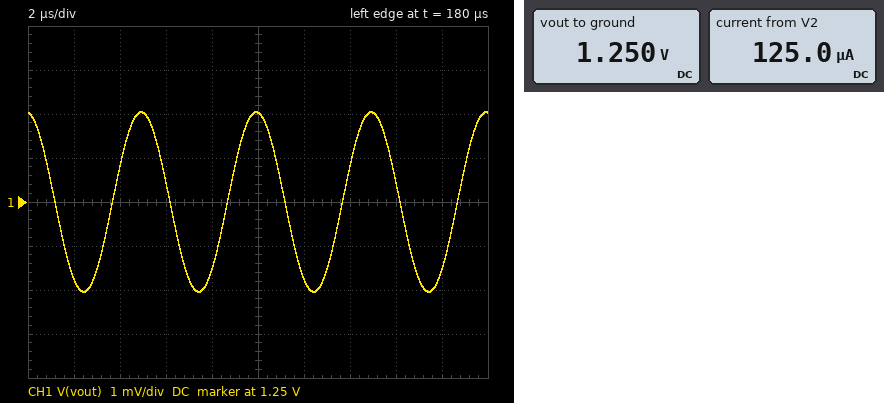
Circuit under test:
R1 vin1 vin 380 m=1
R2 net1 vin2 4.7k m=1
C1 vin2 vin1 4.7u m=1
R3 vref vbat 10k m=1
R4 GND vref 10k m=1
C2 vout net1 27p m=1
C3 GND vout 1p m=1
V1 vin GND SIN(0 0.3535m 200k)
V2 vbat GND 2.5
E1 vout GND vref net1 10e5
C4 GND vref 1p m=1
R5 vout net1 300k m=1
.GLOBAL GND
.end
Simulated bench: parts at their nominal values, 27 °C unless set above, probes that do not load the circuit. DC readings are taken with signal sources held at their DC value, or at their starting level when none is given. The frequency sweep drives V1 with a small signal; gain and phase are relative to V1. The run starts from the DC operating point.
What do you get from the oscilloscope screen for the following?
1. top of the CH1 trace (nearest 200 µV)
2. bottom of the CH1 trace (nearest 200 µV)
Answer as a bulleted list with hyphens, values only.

- 1.2520 V
- 1.2480 V
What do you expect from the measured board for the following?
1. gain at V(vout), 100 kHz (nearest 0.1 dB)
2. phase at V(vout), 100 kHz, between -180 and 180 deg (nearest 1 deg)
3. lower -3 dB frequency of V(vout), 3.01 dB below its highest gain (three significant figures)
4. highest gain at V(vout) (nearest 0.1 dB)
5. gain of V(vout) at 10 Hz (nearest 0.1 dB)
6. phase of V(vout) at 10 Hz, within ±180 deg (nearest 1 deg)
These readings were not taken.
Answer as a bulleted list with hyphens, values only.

- 21.1 dB
- 101 deg
- 6.66 Hz
- 35.4 dB
- 33.8 dB
- -146 deg
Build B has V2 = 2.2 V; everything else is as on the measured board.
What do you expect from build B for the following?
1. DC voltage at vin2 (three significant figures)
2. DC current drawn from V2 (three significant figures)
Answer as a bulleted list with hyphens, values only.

- 1.10 V
- 110 µA
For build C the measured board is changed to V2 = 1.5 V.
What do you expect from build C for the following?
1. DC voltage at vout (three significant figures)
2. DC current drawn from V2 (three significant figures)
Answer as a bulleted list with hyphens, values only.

- 750 mV
- 75.0 µA
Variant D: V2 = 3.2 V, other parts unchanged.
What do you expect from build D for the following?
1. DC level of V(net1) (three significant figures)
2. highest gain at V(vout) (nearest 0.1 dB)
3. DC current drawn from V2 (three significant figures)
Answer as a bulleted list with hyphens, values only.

- 1.60 V
- 35.4 dB
- 160 µA
